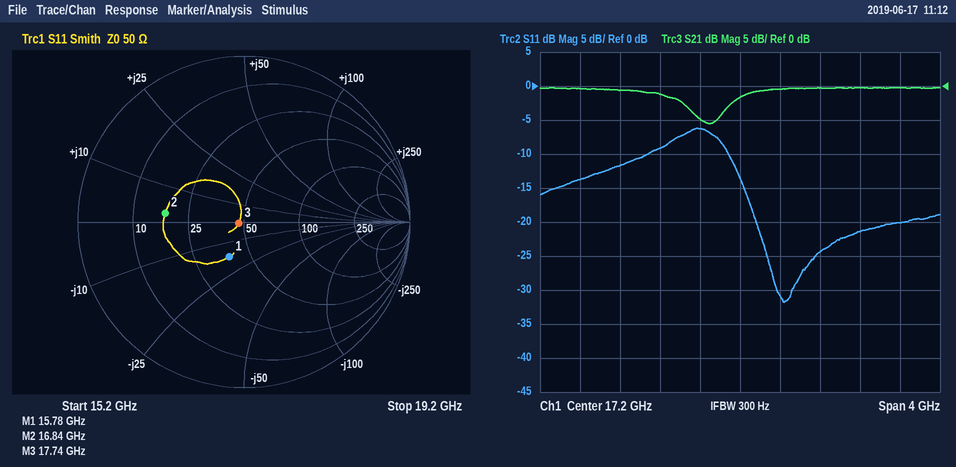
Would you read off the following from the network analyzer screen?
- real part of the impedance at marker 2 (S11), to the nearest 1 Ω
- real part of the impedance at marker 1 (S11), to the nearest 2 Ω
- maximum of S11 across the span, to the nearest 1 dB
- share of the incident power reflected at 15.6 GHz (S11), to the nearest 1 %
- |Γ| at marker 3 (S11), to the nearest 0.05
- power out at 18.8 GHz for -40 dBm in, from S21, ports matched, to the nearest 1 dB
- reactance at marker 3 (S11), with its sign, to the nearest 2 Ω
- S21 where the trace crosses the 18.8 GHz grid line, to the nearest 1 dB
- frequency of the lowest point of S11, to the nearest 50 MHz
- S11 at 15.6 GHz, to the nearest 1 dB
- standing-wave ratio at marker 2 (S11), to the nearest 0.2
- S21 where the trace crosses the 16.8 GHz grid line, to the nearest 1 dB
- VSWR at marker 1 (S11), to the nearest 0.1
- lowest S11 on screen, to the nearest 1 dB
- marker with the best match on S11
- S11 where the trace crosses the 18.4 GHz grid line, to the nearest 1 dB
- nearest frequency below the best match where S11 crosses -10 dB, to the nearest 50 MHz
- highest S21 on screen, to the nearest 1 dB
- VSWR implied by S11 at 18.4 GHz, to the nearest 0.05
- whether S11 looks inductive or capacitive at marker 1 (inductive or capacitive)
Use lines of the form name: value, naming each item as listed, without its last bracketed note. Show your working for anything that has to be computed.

real part of the impedance at marker 2 (S11), to the nearest 1 Ω: 18 Ω
real part of the impedance at marker 1 (S11), to the nearest 2 Ω: 38 Ω
maximum of S11 across the span, to the nearest 1 dB: -6 dB
share of the incident power reflected at 15.6 GHz (S11), to the nearest 1 %: 10^(-14/10) ≈ 4 %
|Γ| at marker 3 (S11), to the nearest 0.05: 0.05
power out at 18.8 GHz for -40 dBm in, from S21, ports matched, to the nearest 1 dB: -40 dBm + (0 dB) = -40 dBm
reactance at marker 3 (S11), with its sign, to the nearest 2 Ω: 0 Ω
S21 where the trace crosses the 18.8 GHz grid line, to the nearest 1 dB: 0 dB
frequency of the lowest point of S11, to the nearest 50 MHz: 17.65 GHz
S11 at 15.6 GHz, to the nearest 1 dB: -14 dB
standing-wave ratio at marker 2 (S11), to the nearest 0.2: 2.8
S21 where the trace crosses the 16.8 GHz grid line, to the nearest 1 dB: -5 dB
VSWR at marker 1 (S11), to the nearest 0.1: 1.6
lowest S11 on screen, to the nearest 1 dB: -32 dB
marker with the best match on S11: marker 3
S11 where the trace crosses the 18.4 GHz grid line, to the nearest 1 dB: -21 dB
nearest frequency below the best match where S11 crosses -10 dB, to the nearest 50 MHz: 17.10 GHz
highest S21 on screen, to the nearest 1 dB: 0 dB
VSWR implied by S11 at 18.4 GHz, to the nearest 0.05: |Γ| = 10^(-21/20) = 0.0891; VSWR = (1 + 0.0891)/(1 − 0.0891) ≈ 1.20
whether S11 looks inductive or capacitive at marker 1: capacitive
